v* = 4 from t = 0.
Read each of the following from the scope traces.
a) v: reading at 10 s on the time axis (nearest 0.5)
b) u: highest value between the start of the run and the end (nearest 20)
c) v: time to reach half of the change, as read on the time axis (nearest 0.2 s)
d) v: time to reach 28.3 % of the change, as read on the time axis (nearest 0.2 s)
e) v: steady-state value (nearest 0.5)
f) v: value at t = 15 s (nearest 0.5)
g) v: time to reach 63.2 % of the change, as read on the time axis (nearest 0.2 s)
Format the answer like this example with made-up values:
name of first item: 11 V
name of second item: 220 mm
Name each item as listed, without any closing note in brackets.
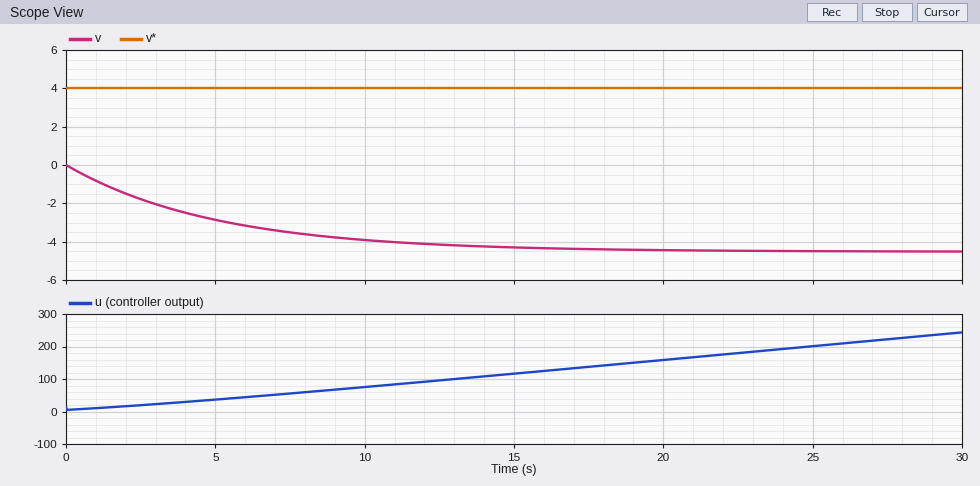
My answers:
v: reading at 10 s on the time axis: -4.0
u: highest value between the start of the run and the end: 240
v: time to reach half of the change, as read on the time axis: 3.4 s
v: time to reach 28.3 % of the change, as read on the time axis: 1.6 s
v: steady-state value: -4.5
v: value at t = 15 s: -4.5
v: time to reach 63.2 % of the change, as read on the time axis: 5.0 s
